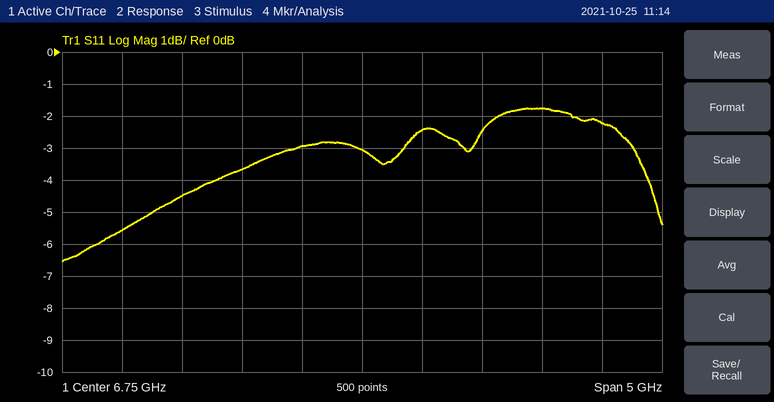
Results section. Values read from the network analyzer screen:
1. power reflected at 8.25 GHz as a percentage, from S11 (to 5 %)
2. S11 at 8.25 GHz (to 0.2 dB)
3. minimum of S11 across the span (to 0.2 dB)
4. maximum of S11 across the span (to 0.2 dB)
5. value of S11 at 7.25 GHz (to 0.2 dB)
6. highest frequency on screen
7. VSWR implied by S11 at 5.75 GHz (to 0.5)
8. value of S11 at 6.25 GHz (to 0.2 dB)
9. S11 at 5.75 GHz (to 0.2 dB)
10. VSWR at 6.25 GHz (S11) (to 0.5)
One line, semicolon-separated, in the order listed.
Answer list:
65 %; -1.8 dB; -6.6 dB; -1.8 dB; -2.4 dB; 9.25 GHz; 5.0; -3.0 dB; -3.6 dB; 6.0
